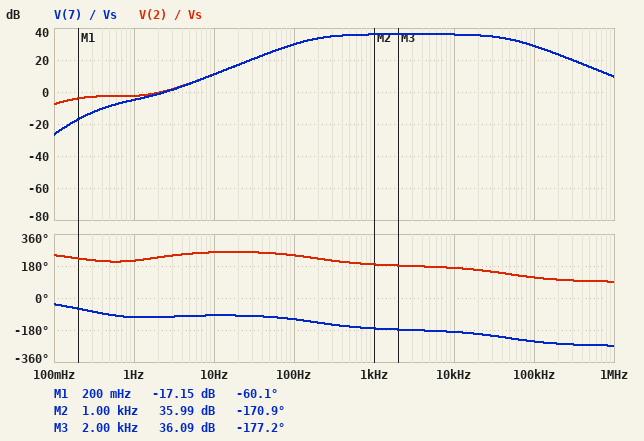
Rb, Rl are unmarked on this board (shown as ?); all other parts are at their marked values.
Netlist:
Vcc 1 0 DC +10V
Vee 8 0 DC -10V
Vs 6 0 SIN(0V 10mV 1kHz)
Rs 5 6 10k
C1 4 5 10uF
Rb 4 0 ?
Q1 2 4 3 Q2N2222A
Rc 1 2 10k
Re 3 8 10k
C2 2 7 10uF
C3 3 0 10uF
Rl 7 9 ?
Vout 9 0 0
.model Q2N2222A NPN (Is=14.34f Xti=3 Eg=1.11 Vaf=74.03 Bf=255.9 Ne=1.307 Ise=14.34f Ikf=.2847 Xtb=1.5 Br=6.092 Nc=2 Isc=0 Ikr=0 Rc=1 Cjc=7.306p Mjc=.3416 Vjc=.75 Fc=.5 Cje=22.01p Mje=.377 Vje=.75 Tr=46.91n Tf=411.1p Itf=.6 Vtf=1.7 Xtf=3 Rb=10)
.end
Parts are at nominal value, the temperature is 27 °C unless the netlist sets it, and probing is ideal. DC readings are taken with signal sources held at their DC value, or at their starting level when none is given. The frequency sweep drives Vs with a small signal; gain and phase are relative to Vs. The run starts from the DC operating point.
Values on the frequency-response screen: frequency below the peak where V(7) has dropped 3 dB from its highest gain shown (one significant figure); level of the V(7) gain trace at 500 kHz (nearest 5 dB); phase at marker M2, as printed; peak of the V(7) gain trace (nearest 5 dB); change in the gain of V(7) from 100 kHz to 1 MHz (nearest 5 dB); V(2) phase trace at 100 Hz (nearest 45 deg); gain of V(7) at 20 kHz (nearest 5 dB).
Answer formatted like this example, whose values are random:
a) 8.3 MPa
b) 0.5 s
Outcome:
a) 200 Hz
b) 15 dB
c) -170.9 deg
d) 35 dB
e) -20 dB
f) 225 deg
g) 35 dB
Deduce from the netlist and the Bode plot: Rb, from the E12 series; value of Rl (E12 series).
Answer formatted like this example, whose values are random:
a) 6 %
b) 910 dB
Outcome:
a) 82 kΩ
b) 18 kΩ
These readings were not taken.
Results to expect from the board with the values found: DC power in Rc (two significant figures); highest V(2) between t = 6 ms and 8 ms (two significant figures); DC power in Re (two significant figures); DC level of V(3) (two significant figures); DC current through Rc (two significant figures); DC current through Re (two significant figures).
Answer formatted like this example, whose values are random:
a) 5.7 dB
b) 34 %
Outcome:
a) 7.8 mW
b) 1.8 V
c) 7.9 mW
d) -1.1 V
e) 880 µA
f) 890 µA
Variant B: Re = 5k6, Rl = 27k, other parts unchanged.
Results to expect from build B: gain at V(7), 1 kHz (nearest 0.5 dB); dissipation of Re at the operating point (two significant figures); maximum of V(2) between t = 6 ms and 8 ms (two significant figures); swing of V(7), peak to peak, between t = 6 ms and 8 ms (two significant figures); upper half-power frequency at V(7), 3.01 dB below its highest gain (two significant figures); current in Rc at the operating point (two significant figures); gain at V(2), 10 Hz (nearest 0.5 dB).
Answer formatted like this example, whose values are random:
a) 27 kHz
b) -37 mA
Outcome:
a) -17.5 dB
b) 9.4 mW
c) -2.7 V
d) 2.7 mV
e) 470 kHz
f) 1.3 mA
g) -17.0 dB
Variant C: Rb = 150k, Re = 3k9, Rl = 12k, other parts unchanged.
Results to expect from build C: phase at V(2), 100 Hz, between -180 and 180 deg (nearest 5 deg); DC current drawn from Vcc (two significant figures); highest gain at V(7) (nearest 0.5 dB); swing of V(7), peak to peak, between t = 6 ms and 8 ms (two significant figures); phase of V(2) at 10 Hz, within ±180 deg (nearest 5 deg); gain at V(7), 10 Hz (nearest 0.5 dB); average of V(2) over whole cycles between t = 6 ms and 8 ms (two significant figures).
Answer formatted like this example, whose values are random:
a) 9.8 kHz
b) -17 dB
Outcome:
a) -170 deg
b) 1.4 mA
c) -16.0 dB
d) 3.1 mV
e) -100 deg
f) -18.0 dB
g) -4.3 V
